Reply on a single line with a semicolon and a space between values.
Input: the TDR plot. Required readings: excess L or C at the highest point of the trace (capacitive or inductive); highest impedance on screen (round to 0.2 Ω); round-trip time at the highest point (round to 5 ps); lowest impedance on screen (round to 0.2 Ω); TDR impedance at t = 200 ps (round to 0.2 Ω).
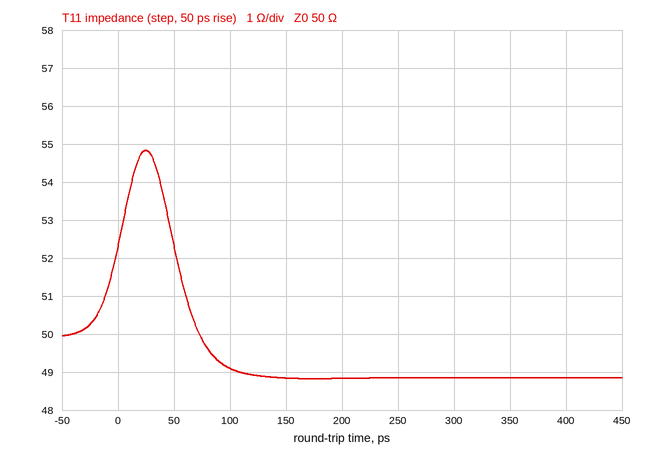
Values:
inductive; 54.8 Ω; 25 ps; 48.8 Ω; 48.8 Ω
